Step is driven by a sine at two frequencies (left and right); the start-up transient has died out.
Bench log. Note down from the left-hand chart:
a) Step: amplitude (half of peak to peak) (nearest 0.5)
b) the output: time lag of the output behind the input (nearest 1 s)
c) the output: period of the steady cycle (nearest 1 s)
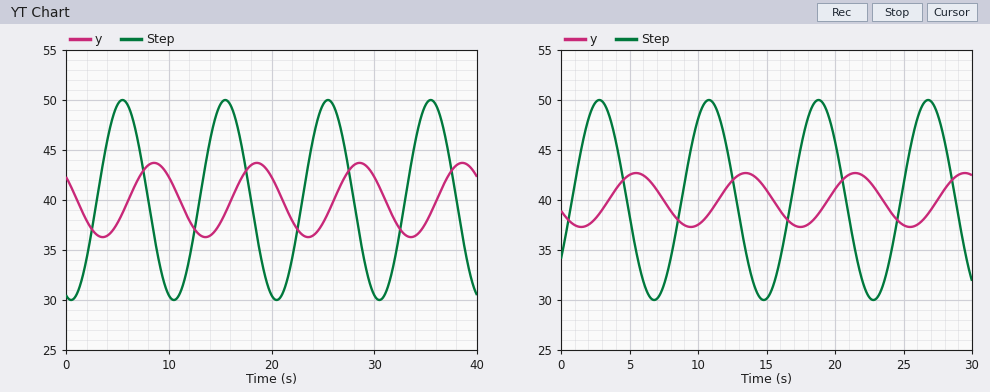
10.0
3 s
10 s
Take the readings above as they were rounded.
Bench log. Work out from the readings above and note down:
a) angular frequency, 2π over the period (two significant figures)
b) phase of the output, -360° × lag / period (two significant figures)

0.63 rad/s
-110°
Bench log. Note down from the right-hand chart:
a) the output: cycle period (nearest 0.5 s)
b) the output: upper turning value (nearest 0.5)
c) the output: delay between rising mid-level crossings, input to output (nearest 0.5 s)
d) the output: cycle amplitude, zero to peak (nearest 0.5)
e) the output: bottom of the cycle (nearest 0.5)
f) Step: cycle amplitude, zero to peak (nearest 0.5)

8.0 s
42.5
2.5 s
2.5
37.5
10.0
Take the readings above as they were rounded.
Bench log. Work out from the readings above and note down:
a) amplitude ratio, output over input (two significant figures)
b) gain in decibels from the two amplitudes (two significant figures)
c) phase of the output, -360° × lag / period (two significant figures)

0.25
-12 dB
-110°
